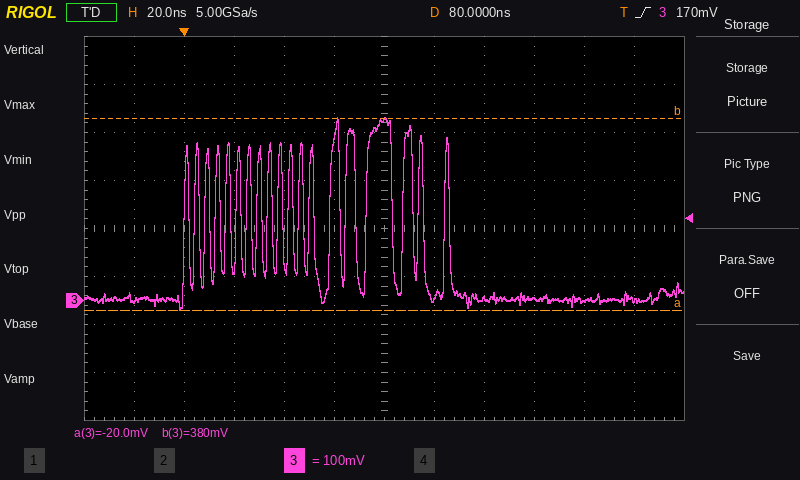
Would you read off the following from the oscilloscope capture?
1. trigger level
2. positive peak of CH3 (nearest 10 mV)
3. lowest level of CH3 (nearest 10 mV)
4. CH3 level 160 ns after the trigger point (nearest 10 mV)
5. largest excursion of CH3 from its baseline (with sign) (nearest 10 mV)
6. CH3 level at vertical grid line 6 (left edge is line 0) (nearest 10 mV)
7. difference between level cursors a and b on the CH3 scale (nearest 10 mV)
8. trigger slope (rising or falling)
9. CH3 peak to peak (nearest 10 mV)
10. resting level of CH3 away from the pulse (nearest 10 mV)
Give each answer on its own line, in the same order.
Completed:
170 mV
380 mV
-20 mV
0 mV
+380 mV
380 mV
400 mV
rising
400 mV
0 mV
